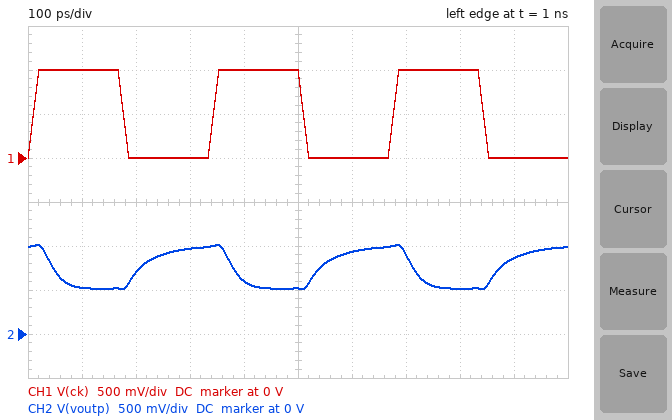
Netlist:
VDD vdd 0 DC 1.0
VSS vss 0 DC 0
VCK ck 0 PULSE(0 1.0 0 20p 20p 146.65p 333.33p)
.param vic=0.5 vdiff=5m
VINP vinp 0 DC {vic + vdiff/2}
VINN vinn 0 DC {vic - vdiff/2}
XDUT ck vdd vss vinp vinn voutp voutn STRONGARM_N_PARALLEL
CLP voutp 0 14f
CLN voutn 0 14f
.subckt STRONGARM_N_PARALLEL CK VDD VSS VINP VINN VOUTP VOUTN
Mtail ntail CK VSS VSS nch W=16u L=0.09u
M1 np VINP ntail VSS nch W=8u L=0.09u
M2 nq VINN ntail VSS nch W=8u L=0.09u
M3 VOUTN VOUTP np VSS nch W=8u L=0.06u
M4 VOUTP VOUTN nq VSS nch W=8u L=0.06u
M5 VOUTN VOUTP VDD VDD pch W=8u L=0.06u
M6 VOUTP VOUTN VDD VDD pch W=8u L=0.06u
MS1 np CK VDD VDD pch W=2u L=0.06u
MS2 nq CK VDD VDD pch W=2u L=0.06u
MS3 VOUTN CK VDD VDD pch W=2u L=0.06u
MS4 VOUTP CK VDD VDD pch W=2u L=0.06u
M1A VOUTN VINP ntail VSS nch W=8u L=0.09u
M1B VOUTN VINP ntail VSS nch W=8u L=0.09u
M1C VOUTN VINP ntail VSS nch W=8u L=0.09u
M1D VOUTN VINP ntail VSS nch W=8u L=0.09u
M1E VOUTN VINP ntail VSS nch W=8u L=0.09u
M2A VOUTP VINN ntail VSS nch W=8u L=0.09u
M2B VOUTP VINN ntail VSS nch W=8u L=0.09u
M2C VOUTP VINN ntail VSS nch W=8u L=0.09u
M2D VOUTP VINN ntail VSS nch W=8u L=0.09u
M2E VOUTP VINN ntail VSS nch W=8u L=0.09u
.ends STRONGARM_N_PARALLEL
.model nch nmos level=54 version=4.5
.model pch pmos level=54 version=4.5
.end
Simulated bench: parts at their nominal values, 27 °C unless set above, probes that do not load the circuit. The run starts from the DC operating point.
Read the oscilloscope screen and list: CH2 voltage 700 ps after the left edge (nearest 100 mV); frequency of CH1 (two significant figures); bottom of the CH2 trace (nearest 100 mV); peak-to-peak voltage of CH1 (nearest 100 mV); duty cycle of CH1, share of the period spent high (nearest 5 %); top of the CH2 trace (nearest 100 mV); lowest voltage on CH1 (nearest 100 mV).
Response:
900 mV
3.0 GHz
500 mV
1.0 V
50 %
1.0 V
0 V
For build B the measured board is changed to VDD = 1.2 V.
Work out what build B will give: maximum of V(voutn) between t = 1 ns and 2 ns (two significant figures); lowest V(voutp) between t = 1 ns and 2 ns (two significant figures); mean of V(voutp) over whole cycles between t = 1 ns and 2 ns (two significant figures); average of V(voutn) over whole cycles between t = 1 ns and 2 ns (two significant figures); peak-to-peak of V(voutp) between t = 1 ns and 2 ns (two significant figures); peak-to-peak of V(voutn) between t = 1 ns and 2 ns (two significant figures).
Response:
1.2 V
690 mV
950 mV
880 mV
520 mV
630 mV
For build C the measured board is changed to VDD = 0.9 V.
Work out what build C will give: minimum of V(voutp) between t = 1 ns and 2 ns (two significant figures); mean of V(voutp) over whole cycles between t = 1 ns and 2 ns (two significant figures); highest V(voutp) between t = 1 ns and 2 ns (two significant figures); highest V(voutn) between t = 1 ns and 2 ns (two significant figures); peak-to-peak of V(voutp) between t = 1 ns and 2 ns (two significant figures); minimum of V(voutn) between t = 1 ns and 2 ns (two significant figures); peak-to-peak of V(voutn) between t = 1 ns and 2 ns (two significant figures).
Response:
420 mV
650 mV
900 mV
850 mV
480 mV
290 mV
560 mV
